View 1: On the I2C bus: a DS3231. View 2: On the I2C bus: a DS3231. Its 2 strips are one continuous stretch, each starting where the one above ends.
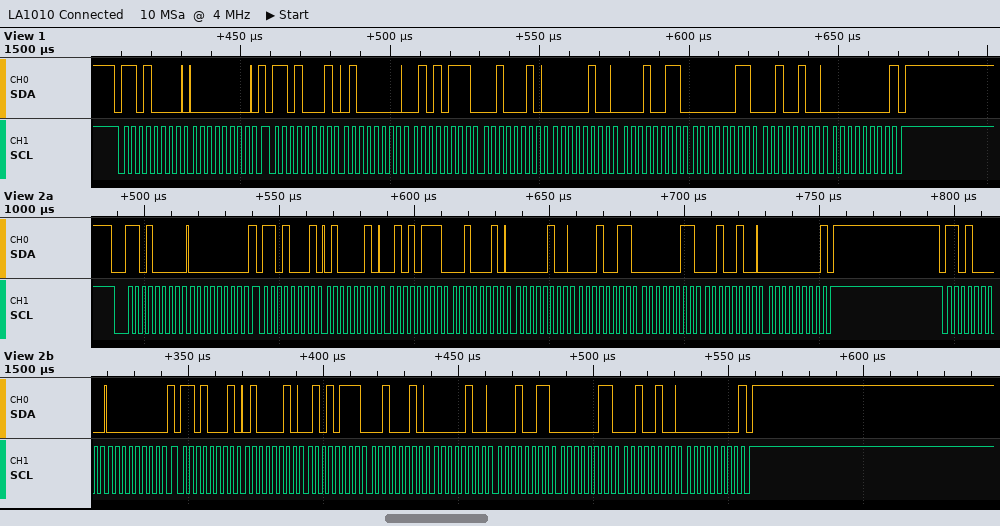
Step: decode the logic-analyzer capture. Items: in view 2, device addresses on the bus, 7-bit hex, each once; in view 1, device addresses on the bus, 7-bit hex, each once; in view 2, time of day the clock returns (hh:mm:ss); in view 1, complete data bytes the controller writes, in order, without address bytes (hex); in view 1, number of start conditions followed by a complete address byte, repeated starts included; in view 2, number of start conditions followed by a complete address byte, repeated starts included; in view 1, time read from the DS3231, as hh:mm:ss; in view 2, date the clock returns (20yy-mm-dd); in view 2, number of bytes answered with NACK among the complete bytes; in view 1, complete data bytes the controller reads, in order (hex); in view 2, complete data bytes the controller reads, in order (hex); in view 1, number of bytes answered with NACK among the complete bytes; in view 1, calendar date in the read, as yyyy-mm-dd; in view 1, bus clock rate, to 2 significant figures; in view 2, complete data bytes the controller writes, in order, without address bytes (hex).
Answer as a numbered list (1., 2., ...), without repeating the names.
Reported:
1. 0x68
2. 0x68
3. 22:57:42
4. 00
5. 2
6. 4
7. 22:57:40
8. 2024-03-13
9. 2
10. 40 57 22 04 13 03 24 00
11. 42 57 22 04 13 03 24 00 42 57 22 04 13 03 24 00
12. 1
13. 2024-03-13
14. 400 kHz
15. 00 00
